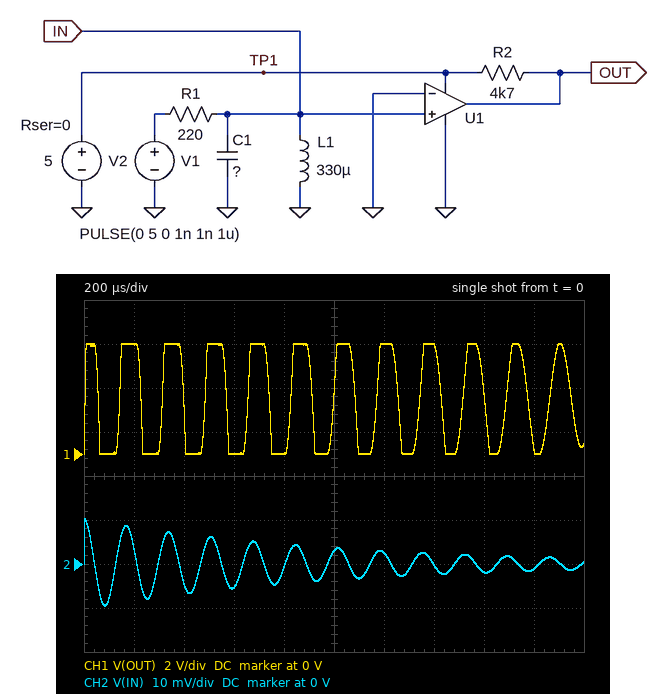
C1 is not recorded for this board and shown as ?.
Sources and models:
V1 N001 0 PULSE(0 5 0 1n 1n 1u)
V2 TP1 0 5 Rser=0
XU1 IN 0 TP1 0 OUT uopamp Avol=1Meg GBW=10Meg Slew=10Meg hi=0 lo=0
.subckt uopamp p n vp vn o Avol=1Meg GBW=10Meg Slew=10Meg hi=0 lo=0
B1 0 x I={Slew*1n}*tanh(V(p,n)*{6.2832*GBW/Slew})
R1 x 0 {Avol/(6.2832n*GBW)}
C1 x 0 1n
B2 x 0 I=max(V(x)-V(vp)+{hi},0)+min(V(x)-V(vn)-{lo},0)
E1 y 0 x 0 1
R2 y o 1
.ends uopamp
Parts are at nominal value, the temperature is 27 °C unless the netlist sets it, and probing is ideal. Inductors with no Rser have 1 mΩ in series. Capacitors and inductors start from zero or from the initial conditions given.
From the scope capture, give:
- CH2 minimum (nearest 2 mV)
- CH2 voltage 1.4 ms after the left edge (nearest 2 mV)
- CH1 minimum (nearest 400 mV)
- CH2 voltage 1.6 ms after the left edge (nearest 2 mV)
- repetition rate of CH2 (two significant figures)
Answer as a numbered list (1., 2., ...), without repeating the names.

1. -10 mV
2. 0 V
3. 0 V
4. -2 mV
5. 5.9 kHz
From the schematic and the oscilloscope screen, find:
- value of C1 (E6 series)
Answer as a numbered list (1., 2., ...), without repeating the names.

1. 2.2 µF
